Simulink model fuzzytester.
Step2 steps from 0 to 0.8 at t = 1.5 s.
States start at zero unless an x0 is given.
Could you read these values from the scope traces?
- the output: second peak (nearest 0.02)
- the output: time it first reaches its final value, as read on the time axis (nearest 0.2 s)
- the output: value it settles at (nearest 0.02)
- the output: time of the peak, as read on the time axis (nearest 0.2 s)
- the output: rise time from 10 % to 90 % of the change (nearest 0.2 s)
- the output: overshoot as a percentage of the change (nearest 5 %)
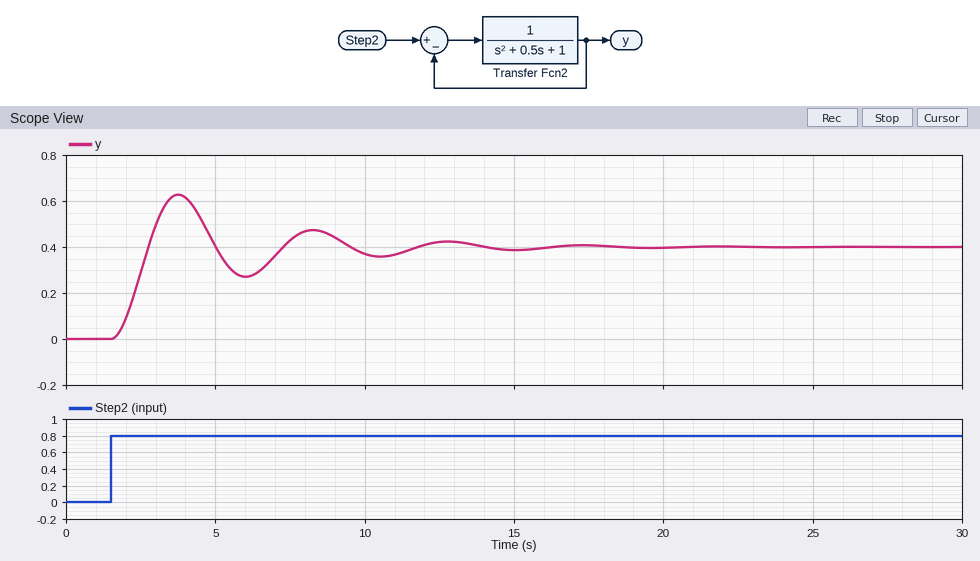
0.48
2.8 s
0.40
3.8 s
0.8 s
55 %
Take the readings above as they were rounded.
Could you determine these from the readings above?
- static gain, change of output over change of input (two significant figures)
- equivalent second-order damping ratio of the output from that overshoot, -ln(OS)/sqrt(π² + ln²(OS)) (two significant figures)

0.50
0.19
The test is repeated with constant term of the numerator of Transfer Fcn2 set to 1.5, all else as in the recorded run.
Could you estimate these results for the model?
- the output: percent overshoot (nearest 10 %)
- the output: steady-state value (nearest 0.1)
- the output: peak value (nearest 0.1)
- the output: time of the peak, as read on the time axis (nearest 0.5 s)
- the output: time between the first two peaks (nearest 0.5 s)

60 %
0.5
0.8
3.5 s
4.0 s
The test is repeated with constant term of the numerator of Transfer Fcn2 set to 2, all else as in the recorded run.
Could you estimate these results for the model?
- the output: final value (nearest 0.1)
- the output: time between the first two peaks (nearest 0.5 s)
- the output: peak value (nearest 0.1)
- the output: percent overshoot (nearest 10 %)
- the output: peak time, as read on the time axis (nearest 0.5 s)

0.5
3.5 s
0.9
60 %
3.5 s
